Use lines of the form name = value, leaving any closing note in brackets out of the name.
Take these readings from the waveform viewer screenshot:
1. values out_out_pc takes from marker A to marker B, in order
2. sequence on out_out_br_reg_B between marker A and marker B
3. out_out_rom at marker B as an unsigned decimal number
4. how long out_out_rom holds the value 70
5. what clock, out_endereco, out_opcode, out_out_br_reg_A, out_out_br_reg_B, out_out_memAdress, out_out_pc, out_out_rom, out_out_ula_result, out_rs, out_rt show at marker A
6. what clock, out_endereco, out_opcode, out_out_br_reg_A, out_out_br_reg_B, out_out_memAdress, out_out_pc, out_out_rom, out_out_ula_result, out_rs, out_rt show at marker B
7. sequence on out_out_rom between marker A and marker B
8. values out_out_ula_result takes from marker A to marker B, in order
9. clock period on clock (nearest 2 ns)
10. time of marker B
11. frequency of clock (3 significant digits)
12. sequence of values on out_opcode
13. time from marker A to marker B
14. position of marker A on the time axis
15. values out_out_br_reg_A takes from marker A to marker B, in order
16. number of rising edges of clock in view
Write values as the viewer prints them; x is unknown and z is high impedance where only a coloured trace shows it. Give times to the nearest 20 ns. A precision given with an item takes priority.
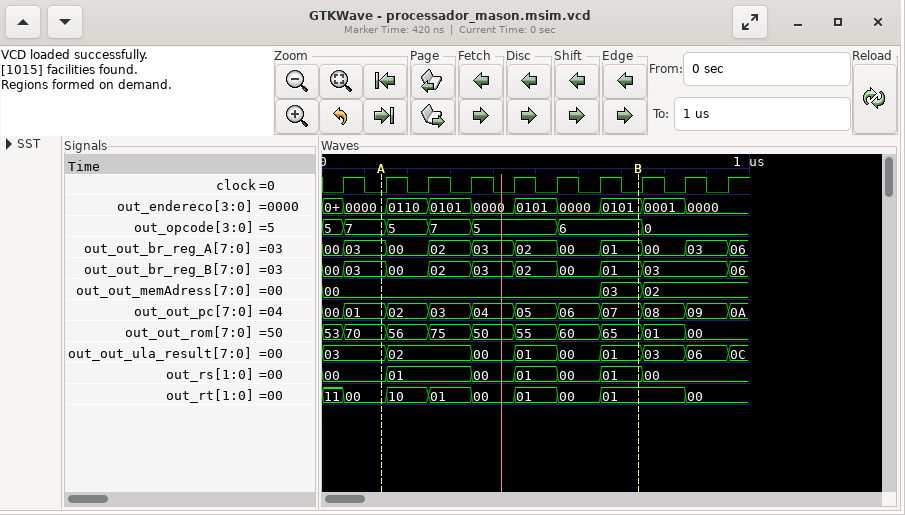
values out_out_pc takes from marker A to marker B, in order = 01, 02, 03, 04, 05, 06, 07
sequence on out_out_br_reg_B between marker A and marker B = 03, 00, 02, 03, 02, 00, 01
out_out_rom at marker B as an unsigned decimal number = 101
how long out_out_rom holds the value 70 = 100 ns
what clock, out_endereco, out_opcode, out_out_br_reg_A, out_out_br_reg_B, out_out_memAdress, out_out_pc, out_out_rom, out_out_ula_result, out_rs, out_rt show at marker A = clock=0, out_endereco=0000, out_opcode=7, out_out_br_reg_A=03, out_out_br_reg_B=03, out_out_memAdress=00, out_out_pc=01, out_out_rom=70, out_out_ula_result=03, out_rs=00, out_rt=00
what clock, out_endereco, out_opcode, out_out_br_reg_A, out_out_br_reg_B, out_out_memAdress, out_out_pc, out_out_rom, out_out_ula_result, out_rs, out_rt show at marker B = clock=0, out_endereco=0101, out_opcode=6, out_out_br_reg_A=01, out_out_br_reg_B=01, out_out_memAdress=03, out_out_pc=07, out_out_rom=65, out_out_ula_result=01, out_rs=01, out_rt=01
sequence on out_out_rom between marker A and marker B = 70, 56, 75, 50, 55, 60, 65
values out_out_ula_result takes from marker A to marker B, in order = 03, 02, 00, 01, 00, 01
clock period on clock = 100 ns
time of marker B = 740 ns
frequency of clock = 10.0 MHz
sequence of values on out_opcode = 5, 7, 5, 7, 5, 6, 0
time from marker A to marker B = 600 ns
position of marker A on the time axis = 140 ns
values out_out_br_reg_A takes from marker A to marker B, in order = 03, 00, 02, 03, 02, 00, 01
number of rising edges of clock in view = 10
